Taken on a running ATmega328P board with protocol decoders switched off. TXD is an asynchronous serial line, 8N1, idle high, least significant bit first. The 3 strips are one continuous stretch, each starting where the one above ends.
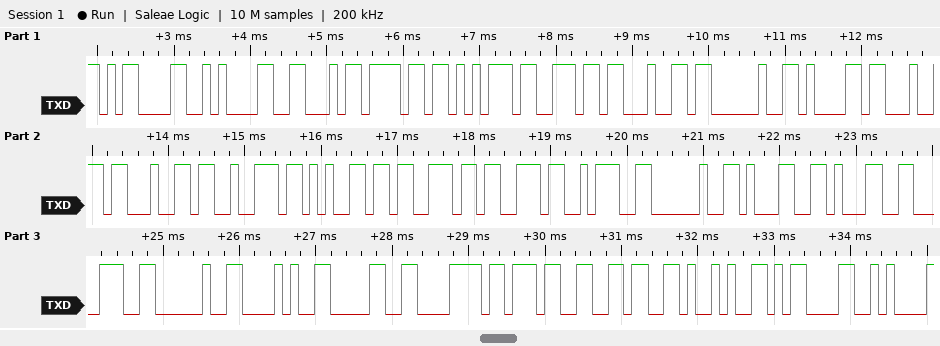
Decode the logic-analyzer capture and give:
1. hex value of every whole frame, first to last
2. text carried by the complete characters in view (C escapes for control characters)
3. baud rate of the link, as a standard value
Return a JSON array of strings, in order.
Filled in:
["0x0D 0x0A 0x46 0x6F 0x75 0x6E 0x64 0x20 0x61 0x64 0x64 0x72 0x65 0x73 0x73 0x3A 0x20 0x31 0x31 0x38 0x20 0x28 0x30 0x78 0x37 0x36 0x29 0x0D 0x0A", "\"\\r\\nFound address: 118 (0x76)\\r\\n\"", "9600 baud"]
